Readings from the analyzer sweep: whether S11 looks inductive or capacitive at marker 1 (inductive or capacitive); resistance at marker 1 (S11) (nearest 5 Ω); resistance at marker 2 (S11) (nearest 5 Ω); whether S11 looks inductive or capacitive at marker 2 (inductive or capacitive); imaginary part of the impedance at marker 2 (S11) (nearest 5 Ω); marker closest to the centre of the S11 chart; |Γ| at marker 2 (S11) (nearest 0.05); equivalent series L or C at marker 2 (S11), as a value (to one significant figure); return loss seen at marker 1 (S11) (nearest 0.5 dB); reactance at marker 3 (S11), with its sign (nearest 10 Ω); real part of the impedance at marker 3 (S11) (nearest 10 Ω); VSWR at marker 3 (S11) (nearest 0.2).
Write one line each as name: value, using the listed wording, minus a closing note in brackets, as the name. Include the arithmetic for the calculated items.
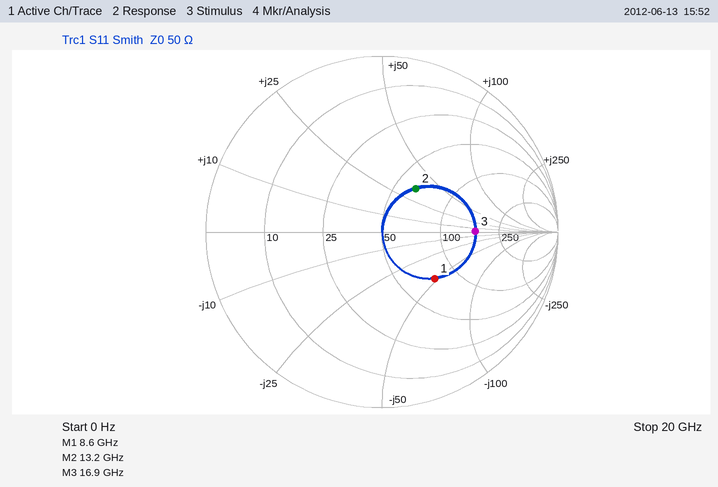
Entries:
whether S11 looks inductive or capacitive at marker 1: capacitive
resistance at marker 1 (S11): 75 Ω
resistance at marker 2 (S11): 65 Ω
whether S11 looks inductive or capacitive at marker 2: inductive
imaginary part of the impedance at marker 2 (S11): +35 Ω
marker closest to the centre of the S11 chart: marker 2
|Γ| at marker 2 (S11): 0.30
equivalent series L or C at marker 2 (S11), as a value: L = 35 Ω/(2π × 13.2 GHz) ≈ 422 pH, so 400 pH to one significant figure
return loss seen at marker 1 (S11): 8.0 dB
reactance at marker 3 (S11), with its sign: 0 Ω
real part of the impedance at marker 3 (S11): 160 Ω
VSWR at marker 3 (S11): 3.2
